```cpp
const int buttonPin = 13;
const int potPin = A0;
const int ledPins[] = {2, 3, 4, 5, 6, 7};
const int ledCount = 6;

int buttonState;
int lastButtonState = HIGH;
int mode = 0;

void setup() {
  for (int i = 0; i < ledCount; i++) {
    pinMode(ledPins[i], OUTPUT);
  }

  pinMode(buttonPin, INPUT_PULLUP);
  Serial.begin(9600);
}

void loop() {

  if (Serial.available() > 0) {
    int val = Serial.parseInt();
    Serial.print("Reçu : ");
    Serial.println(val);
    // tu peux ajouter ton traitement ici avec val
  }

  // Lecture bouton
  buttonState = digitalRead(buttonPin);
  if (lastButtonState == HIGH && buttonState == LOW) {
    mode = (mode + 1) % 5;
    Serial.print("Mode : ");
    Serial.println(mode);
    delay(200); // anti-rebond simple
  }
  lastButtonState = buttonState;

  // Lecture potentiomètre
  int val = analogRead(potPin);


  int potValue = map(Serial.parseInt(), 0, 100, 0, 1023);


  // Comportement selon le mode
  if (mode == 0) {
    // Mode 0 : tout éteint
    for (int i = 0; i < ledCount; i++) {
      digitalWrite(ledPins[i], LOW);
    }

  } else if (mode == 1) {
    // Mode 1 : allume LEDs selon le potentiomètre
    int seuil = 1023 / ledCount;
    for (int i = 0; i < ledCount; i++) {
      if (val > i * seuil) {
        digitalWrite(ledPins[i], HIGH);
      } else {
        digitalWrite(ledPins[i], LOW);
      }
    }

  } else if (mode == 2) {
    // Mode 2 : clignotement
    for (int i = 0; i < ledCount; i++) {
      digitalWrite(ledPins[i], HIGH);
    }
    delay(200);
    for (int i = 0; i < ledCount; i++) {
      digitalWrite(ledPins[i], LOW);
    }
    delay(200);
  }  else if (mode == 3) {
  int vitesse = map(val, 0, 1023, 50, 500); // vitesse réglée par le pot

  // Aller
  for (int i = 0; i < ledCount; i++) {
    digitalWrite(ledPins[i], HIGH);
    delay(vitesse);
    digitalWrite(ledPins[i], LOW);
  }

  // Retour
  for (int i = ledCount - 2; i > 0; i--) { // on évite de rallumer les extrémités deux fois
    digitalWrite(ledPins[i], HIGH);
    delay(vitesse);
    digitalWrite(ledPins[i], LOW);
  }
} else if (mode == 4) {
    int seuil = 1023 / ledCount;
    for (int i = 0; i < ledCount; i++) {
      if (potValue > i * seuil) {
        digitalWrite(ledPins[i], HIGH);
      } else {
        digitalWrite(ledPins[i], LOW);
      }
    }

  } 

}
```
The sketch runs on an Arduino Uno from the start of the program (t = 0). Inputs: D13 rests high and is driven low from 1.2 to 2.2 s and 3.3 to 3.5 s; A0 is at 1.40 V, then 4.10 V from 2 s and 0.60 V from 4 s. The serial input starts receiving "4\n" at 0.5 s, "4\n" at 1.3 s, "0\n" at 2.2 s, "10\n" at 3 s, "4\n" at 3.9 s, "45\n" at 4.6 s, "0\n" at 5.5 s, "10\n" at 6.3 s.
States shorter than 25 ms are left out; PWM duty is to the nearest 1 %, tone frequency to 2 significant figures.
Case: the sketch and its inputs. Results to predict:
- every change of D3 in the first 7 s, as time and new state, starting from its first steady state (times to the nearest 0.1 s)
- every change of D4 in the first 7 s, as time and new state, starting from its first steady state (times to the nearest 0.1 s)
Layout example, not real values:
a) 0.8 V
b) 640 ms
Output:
a) 0 s low; 2.2 s high; 5.5 s low
b) 0 s low; 3.9 s high; 5.5 s low
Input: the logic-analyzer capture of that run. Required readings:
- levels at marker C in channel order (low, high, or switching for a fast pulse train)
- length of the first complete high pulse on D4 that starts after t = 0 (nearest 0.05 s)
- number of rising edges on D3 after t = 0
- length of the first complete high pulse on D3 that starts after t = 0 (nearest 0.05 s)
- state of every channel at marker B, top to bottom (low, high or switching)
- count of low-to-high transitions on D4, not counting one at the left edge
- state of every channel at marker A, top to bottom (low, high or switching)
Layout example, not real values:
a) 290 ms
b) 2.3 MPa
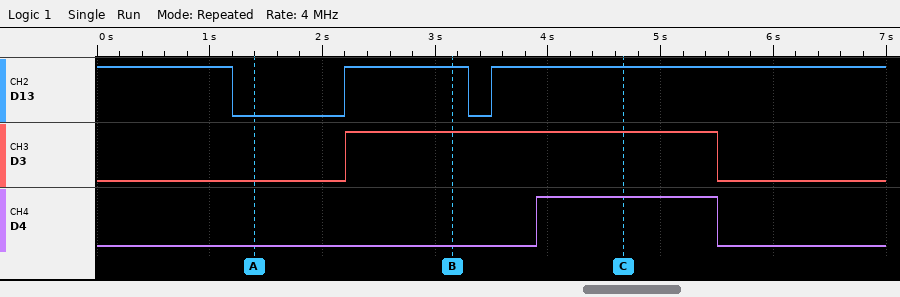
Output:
a) D13 high, D3 high, D4 high
b) 1.60 s
c) 1
d) 3.30 s
e) D13 high, D3 high, D4 low
f) 1
g) D13 low, D3 low, D4 low
